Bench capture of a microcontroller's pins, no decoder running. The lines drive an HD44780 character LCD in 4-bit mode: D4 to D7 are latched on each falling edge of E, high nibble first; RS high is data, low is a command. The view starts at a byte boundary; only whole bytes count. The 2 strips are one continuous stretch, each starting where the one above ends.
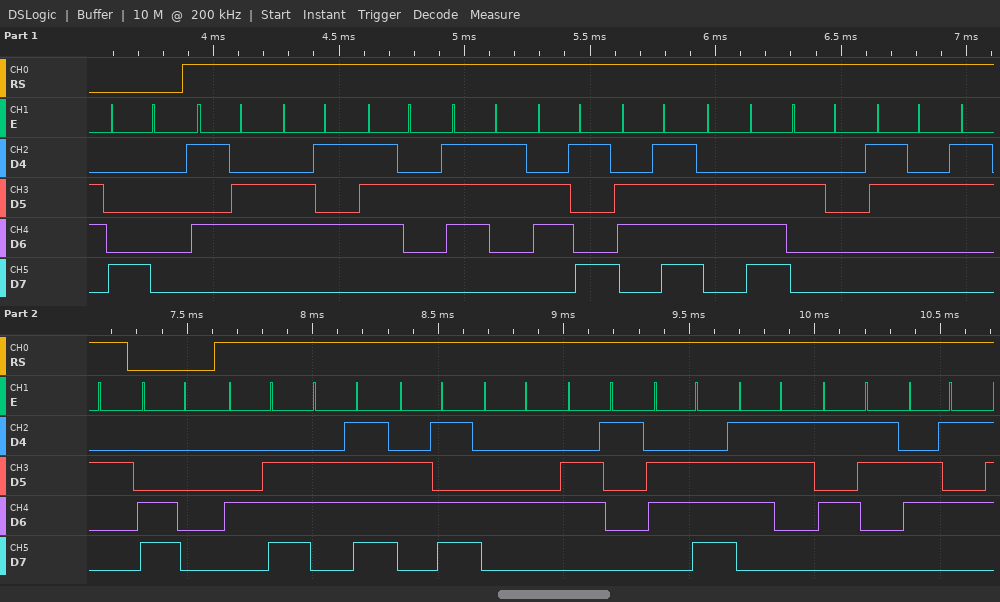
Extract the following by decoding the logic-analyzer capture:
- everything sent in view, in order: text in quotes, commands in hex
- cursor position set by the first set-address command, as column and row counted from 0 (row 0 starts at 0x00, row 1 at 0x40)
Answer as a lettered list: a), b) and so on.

a) 0x80 "Version 22" 0xC0 "NomDansSe"
b) column 0, row 0
